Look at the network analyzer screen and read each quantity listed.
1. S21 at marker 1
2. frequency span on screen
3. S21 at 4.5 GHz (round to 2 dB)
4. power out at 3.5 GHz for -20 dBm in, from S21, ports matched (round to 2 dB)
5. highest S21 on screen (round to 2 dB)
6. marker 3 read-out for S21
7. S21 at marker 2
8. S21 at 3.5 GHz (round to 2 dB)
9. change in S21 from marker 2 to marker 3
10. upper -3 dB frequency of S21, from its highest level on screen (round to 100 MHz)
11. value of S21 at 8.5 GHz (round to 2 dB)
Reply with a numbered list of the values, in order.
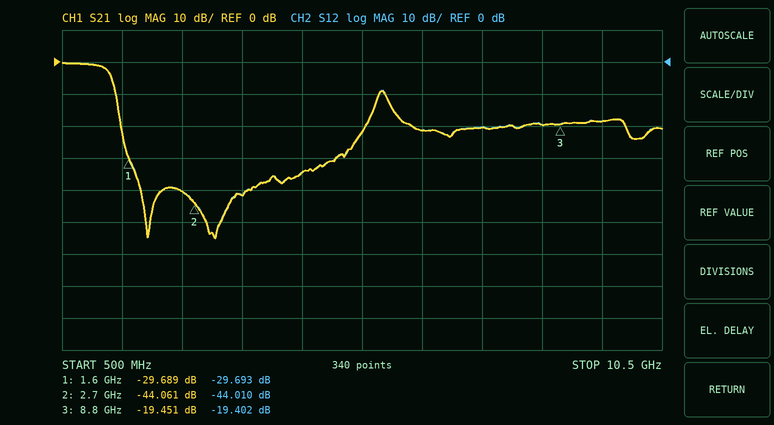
1. -29.689 dB
2. 10 GHz
3. -34 dB
4. -62 dBm
5. 0 dB
6. -19.451 dB
7. -44.061 dB
8. -42 dB
9. 24.610 dB
10. 1.3 GHz
11. -20 dB
